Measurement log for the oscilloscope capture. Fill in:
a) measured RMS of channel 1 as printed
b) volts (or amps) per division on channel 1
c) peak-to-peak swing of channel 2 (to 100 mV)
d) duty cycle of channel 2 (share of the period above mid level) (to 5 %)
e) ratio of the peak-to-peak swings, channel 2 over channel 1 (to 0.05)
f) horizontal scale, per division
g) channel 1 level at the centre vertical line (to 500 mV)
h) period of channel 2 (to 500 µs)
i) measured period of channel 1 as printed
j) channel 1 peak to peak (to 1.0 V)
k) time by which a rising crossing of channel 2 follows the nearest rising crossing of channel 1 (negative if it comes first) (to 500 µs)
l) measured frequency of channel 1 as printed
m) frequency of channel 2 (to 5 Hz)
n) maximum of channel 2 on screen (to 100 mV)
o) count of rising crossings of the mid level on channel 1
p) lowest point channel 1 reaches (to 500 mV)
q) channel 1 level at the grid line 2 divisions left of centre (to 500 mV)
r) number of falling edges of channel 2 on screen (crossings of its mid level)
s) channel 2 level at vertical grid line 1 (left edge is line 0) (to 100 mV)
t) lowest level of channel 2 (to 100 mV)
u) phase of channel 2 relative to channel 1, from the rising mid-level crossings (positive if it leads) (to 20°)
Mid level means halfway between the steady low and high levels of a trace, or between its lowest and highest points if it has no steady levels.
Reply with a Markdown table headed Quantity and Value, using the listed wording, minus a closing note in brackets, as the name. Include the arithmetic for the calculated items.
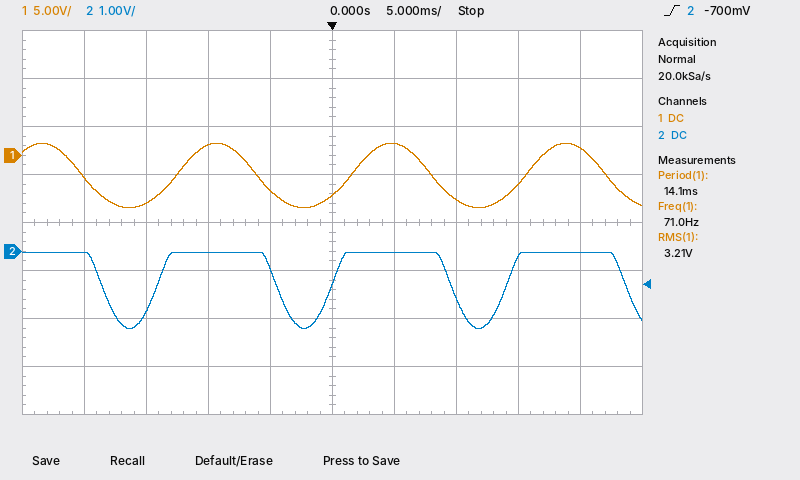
| Quantity | Value |
|---|---|
| measured RMS of channel 1 as printed | 3.21 V |
| volts (or amps) per division on channel 1 | 5 V |
| peak-to-peak swing of channel 2 | 0.0 V − (-1.6 V) = 1.6 V |
| duty cycle of channel 2 (share of the period above mid level) | 70 % |
| ratio of the peak-to-peak swings, channel 2 over channel 1 | 1.6 V / 7.0 V ≈ 0.229, so 0.25 to the nearest 0.05 |
| horizontal scale, per division | 5 ms |
| channel 1 level at the centre vertical line | -4.0 V |
| period of channel 2 | 14.0 ms |
| measured period of channel 1 as printed | 14.1 ms |
| channel 1 peak to peak | 7.0 V |
| time by which a rising crossing of channel 2 follows the nearest rising crossing of channel 1 (negative if it comes first) | -1.5 ms |
| measured frequency of channel 1 as printed | 71.0 Hz |
| frequency of channel 2 | 1 / 14.0 ms ≈ 71.4 Hz, so 70 Hz to the nearest 5 Hz |
| maximum of channel 2 on screen | 0.0 V |
| count of rising crossings of the mid level on channel 1 | 3 |
| lowest point channel 1 reaches | -5.5 V |
| channel 1 level at the grid line 2 divisions left of centre | 1.0 V |
| number of falling edges of channel 2 on screen | 4 |
| channel 2 level at vertical grid line 1 (left edge is line 0) | 0.0 V |
| lowest level of channel 2 | -1.6 V |
| phase of channel 2 relative to channel 1, from the rising mid-level crossings (positive if it leads) | −360° × (-1.5 ms) / 14.0 ms ≈ +38.6°, so +40° to the nearest 20° |
